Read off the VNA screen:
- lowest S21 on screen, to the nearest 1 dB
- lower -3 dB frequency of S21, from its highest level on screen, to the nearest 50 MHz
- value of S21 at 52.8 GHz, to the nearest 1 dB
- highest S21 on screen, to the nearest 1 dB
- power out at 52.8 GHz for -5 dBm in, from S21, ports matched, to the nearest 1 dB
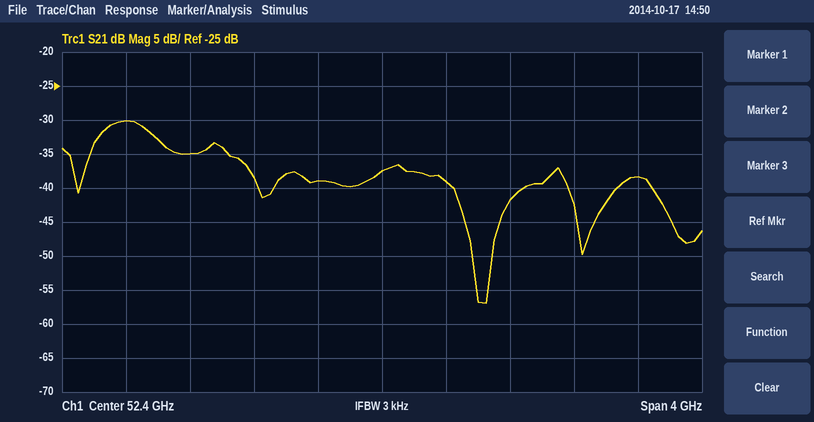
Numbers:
-57 dB
50.60 GHz
-39 dB
-30 dB
-44 dBm
